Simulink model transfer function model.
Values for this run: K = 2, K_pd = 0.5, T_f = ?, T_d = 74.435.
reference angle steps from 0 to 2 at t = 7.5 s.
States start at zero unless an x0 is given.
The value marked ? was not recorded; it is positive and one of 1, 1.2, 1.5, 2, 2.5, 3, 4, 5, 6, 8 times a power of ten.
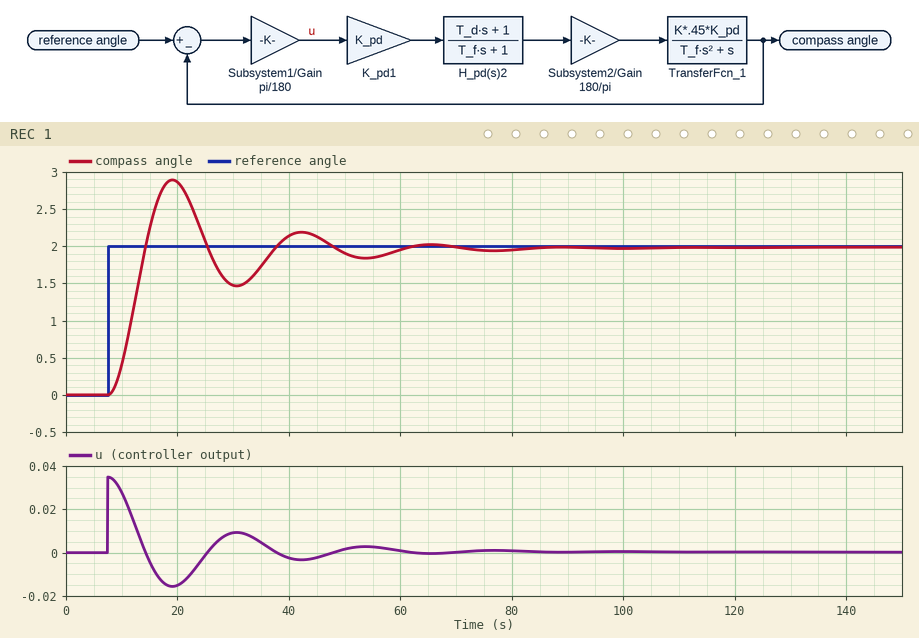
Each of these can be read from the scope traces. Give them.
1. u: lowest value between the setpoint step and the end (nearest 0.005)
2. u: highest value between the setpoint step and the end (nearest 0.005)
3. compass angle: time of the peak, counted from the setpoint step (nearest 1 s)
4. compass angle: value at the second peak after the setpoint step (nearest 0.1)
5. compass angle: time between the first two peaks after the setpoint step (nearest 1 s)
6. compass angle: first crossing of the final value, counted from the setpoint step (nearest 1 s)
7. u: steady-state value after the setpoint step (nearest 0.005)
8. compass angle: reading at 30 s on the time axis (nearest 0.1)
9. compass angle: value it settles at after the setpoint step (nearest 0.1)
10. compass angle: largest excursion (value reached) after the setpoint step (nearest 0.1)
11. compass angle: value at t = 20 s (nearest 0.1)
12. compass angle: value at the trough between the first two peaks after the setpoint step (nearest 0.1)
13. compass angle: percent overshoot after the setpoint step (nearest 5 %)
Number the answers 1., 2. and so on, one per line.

1. -0.015
2. 0.035
3. 12 s
4. 2.2
5. 23 s
6. 7 s
7. 0.000
8. 1.5
9. 2.0
10. 2.9
11. 2.9
12. 1.5
13. 45 %
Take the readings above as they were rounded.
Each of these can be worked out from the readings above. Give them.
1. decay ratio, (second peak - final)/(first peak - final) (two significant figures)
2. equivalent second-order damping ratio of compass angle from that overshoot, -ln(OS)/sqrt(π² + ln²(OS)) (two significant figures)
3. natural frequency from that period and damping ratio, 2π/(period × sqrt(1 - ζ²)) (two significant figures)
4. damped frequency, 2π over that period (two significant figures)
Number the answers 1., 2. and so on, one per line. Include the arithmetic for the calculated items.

1. (2.2 - 2) / (2.9 - 2) = 0.22
2. ln(0.45) = -0.799; 0.799 / sqrt(9.870 + 0.638) = 0.25
3. 2π / (23 × sqrt(1 - 0.25²)) = 0.28 rad/s
4. 2π / 23 = 0.27 rad/s
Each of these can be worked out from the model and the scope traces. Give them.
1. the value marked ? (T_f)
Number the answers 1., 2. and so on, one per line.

1. 15
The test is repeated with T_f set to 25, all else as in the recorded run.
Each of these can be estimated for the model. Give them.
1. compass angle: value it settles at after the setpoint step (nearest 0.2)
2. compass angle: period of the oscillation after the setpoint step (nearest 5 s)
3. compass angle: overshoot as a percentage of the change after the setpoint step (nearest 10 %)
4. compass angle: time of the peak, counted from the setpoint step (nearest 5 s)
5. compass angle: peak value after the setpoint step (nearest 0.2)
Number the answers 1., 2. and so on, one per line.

1. 2.0
2. 40 s
3. 50 %
4. 20 s
5. 3.0
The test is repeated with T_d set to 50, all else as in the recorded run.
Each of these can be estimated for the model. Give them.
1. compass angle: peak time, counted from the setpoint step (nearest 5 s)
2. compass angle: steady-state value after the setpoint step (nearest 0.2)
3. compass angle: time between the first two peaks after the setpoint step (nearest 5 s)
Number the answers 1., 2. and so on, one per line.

1. 15 s
2. 2.0
3. 30 s
